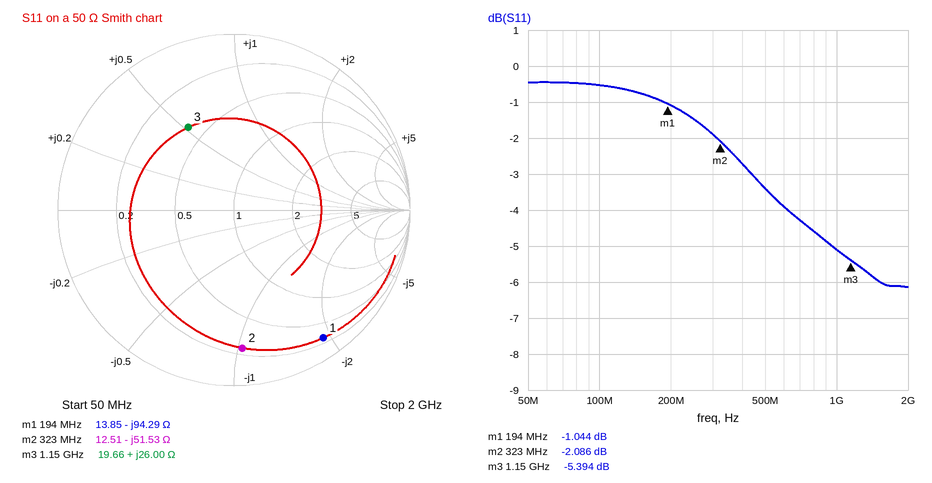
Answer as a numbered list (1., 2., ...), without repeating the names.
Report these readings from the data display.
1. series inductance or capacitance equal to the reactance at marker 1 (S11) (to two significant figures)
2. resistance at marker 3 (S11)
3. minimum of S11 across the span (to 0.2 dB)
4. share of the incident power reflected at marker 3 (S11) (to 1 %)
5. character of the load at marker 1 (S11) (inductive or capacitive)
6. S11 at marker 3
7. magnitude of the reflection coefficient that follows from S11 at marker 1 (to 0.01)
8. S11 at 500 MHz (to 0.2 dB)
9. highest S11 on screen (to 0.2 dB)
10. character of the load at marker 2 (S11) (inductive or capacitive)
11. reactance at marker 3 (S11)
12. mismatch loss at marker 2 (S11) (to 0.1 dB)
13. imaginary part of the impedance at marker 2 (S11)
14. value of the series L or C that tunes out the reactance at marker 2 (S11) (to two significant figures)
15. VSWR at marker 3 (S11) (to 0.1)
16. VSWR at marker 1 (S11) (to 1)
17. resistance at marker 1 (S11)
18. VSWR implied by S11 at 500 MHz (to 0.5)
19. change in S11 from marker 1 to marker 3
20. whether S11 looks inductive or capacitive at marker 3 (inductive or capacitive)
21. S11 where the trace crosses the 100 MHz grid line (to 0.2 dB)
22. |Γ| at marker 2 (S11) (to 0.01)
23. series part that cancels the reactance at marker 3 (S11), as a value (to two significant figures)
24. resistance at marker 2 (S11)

1. 8.7 pF
2. 19.66 Ω
3. -6.2 dB
4. 29 %
5. capacitive
6. -5.394 dB
7. 0.89
8. -3.4 dB
9. -0.4 dB
10. capacitive
11. +26.00 Ω
12. 4.2 dB
13. -51.53 Ω
14. 25 nH
15. 3.3
16. 17
17. 13.85 Ω
18. 5.0
19. -4.350 dB
20. inductive
21. -0.6 dB
22. 0.79
23. 5.3 pF
24. 12.51 Ω
